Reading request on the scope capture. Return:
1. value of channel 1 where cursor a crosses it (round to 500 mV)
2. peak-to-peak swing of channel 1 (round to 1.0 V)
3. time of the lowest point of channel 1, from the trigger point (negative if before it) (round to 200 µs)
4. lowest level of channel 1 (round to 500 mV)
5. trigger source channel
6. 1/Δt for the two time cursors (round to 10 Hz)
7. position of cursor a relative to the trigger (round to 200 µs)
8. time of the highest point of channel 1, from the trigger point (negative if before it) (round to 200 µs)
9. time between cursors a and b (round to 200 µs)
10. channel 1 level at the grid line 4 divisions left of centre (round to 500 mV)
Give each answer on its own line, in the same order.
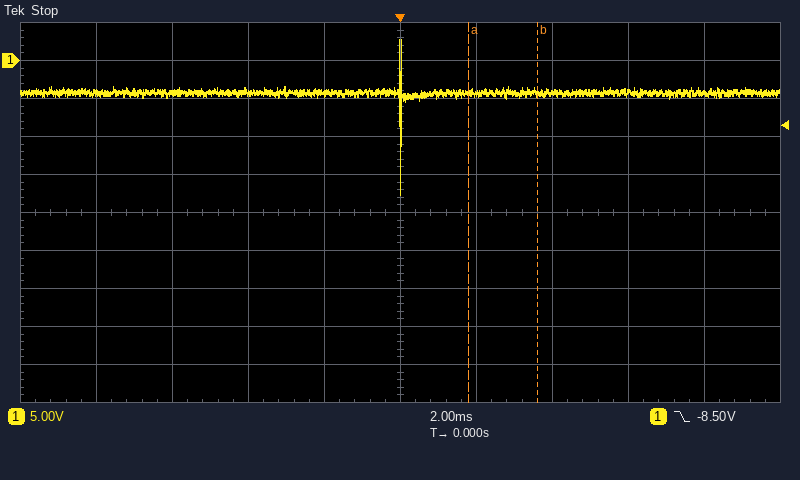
-4.0 V
20.0 V
0.0 ms
-17.5 V
channel 1
560 Hz
+1.8 ms
0.0 ms
1.8 ms
-4.5 V
